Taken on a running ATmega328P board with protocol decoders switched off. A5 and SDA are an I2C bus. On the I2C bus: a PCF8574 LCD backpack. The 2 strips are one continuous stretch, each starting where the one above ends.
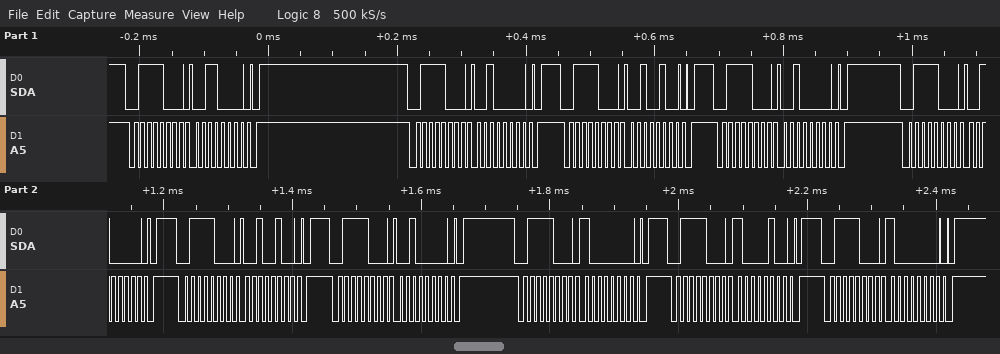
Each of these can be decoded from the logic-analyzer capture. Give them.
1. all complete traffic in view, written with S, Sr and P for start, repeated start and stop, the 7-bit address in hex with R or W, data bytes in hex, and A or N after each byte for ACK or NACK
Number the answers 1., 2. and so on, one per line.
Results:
1. S 3CW A 30 A P S 3CW A 20 A P S 3CW A 24 A P S 3CW A 20 A P S 3CW A 20 A P S 3CW A 24 A P S 3CW A 20 A P S 3CW A 80 A P S 3CW A 84 A P S 3CW A 80 A P
